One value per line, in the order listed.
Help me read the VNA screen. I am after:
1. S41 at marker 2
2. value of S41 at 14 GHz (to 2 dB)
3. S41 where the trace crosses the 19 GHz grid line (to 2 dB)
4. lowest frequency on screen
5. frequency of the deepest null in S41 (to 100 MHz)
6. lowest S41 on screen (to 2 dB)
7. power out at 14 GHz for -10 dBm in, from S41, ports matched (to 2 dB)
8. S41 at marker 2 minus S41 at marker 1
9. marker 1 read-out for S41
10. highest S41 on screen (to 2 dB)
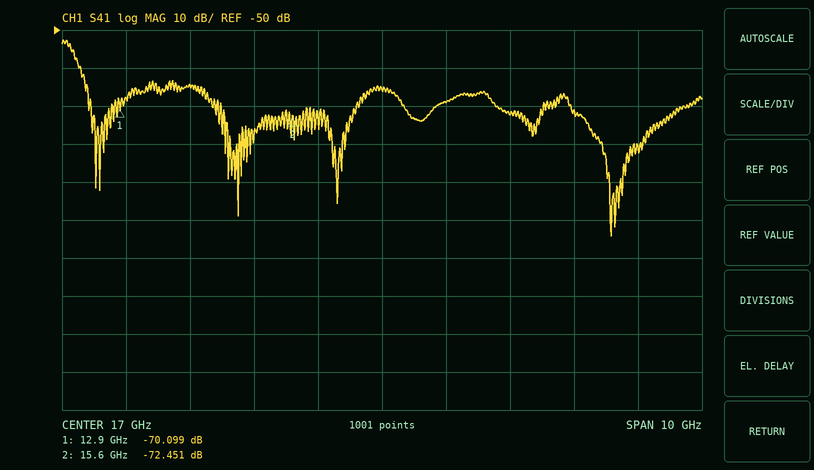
-72.451 dB
-64 dB
-72 dB
12 GHz
20.6 GHz
-104 dB
-74 dBm
-2.352 dB
-70.099 dB
-52 dB
